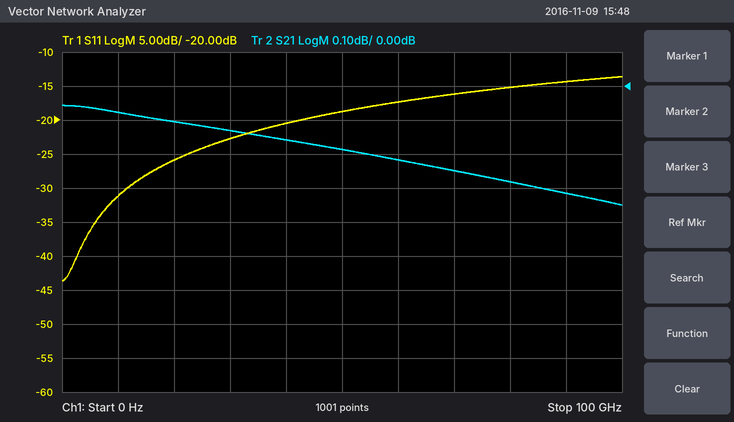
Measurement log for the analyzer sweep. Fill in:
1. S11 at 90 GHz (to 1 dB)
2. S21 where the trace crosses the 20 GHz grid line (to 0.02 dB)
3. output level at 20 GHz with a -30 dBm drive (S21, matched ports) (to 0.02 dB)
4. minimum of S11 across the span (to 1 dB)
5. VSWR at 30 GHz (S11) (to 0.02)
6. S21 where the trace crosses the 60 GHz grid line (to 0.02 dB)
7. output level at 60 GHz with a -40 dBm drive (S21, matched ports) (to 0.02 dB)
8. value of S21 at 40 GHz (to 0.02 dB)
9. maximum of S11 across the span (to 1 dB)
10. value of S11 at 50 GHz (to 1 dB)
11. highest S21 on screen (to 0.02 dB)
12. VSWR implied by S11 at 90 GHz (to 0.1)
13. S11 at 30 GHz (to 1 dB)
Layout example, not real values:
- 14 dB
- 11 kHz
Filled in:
- -14 dB
- -0.10 dB
- -30.10 dBm
- -44 dB
- 1.16
- -0.22 dB
- -40.22 dBm
- -0.16 dB
- -14 dB
- -19 dB
- -0.06 dB
- 1.5
- -23 dB
